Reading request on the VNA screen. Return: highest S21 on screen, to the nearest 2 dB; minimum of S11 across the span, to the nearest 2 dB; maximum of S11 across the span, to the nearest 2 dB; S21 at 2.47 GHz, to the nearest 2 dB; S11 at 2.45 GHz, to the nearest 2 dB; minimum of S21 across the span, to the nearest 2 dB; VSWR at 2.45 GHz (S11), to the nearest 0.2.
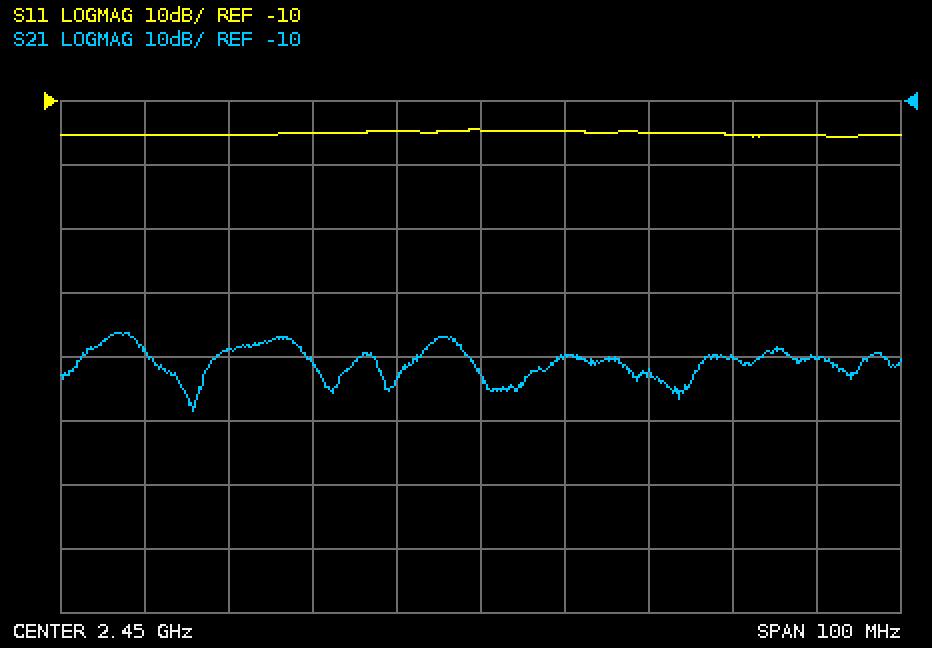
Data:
-46 dB
-16 dB
-14 dB
-52 dB
-14 dB
-58 dB
1.4
